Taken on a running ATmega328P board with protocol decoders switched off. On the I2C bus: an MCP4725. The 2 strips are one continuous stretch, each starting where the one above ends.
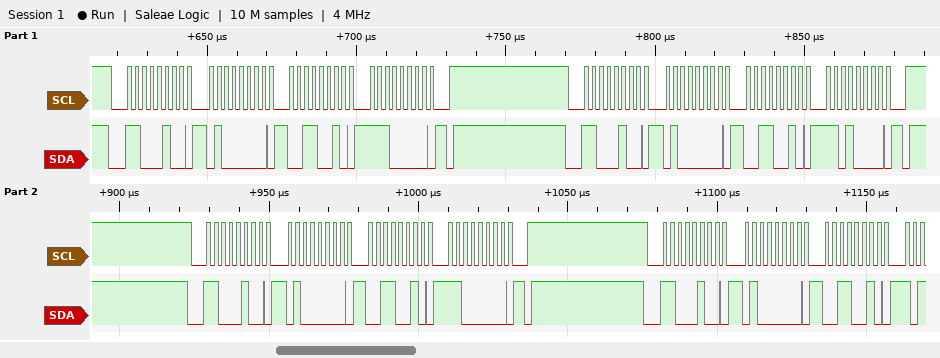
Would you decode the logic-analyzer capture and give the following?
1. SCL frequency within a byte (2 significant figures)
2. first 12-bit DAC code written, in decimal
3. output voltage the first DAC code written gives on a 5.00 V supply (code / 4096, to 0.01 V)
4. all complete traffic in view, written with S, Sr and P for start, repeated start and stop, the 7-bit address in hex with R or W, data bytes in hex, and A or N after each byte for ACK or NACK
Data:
400 kHz
814
0.99 V
S 62W A 40 A 32 A E0 A P S 62W A 40 A 32 A D0 A P S 62W A 40 A 32 A C0 A P S 62W A 40 A 32 A
